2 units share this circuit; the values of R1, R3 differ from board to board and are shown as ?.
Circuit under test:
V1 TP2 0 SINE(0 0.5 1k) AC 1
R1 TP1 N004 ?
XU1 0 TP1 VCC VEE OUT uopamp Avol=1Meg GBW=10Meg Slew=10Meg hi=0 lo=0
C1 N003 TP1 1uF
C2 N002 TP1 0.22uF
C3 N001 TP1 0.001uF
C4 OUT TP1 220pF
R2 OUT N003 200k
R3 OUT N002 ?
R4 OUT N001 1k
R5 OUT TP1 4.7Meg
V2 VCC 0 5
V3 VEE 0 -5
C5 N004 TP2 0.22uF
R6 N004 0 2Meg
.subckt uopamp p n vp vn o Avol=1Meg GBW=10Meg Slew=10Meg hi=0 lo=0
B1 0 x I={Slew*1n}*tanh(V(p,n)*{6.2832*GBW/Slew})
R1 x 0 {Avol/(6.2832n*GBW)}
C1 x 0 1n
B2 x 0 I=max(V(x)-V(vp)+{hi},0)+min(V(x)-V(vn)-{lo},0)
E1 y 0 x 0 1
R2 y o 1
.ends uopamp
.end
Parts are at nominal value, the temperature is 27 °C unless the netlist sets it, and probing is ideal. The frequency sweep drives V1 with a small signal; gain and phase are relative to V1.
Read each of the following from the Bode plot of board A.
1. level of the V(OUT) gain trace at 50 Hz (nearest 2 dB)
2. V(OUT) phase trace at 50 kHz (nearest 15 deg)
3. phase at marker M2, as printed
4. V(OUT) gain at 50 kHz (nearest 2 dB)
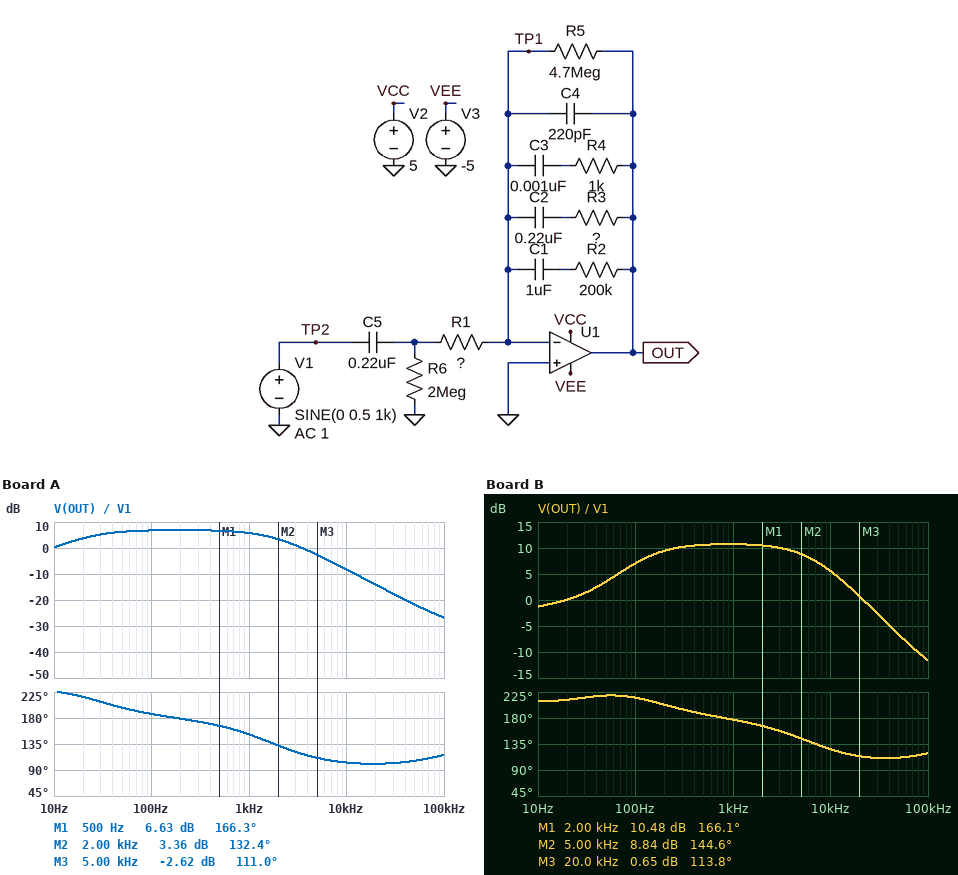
6 dB
105 deg
132.4 deg
-22 dB
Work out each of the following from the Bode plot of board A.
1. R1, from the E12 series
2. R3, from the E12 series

33 kΩ
120 kΩ
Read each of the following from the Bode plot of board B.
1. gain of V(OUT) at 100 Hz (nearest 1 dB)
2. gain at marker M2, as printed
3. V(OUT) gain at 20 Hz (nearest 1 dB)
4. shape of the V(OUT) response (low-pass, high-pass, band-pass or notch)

7 dB
8.84 dB
0 dB
band-pass
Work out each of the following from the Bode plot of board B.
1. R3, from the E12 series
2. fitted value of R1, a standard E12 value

22 kΩ
5.6 kΩ
